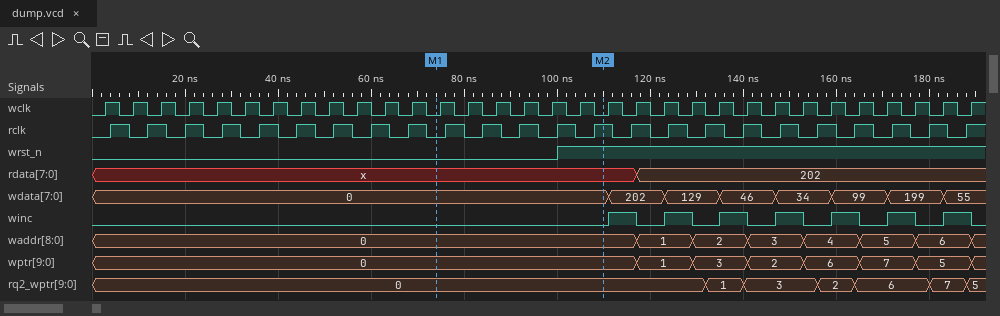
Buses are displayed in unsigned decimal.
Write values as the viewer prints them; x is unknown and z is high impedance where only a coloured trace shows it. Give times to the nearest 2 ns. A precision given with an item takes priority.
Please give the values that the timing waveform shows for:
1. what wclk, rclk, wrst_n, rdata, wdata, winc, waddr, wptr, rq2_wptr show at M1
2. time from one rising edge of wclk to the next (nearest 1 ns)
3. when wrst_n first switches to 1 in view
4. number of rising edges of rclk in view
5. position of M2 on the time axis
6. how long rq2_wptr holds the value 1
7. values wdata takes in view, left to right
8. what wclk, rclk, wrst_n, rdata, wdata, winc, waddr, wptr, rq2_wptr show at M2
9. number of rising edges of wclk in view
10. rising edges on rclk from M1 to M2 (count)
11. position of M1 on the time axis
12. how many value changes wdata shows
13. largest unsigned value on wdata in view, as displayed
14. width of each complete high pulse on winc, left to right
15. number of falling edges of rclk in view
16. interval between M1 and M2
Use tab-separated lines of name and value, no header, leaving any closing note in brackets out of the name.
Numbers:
what wclk, rclk, wrst_n, rdata, wdata, winc, waddr, wptr, rq2_wptr show at M1	wclk=0, rclk=0, wrst_n=0, rdata=x, wdata=0, winc=0, waddr=0, wptr=0, rq2_wptr=0
time from one rising edge of wclk to the next	6 ns
when wrst_n first switches to 1 in view	100 ns
number of rising edges of rclk in view	24
position of M2 on the time axis	110 ns
how long rq2_wptr holds the value 1	8 ns
values wdata takes in view, left to right	0, 202, 129, 46, 34, 99, 199, 55
what wclk, rclk, wrst_n, rdata, wdata, winc, waddr, wptr, rq2_wptr show at M2	wclk=0, rclk=1, wrst_n=1, rdata=x, wdata=0, winc=0, waddr=0, wptr=0, rq2_wptr=0
number of rising edges of wclk in view	32
rising edges on rclk from M1 to M2	5
position of M1 on the time axis	74 ns
how many value changes wdata shows	7
largest unsigned value on wdata in view, as displayed	202
width of each complete high pulse on winc, left to right	6 ns, 6 ns, 6 ns, 6 ns, 6 ns, 6 ns, 6 ns
number of falling edges of rclk in view	23
interval between M1 and M2	36 ns
